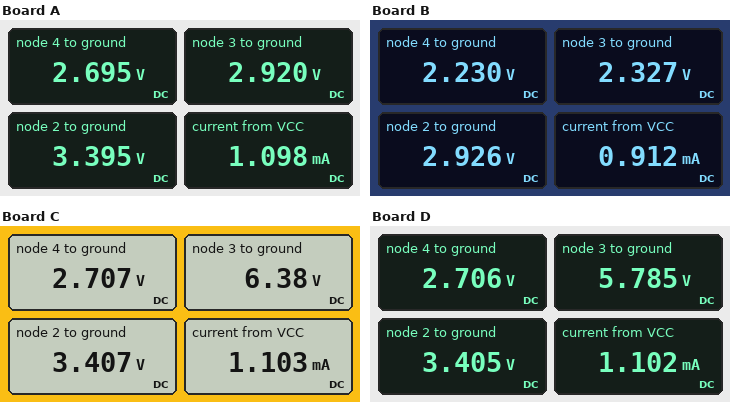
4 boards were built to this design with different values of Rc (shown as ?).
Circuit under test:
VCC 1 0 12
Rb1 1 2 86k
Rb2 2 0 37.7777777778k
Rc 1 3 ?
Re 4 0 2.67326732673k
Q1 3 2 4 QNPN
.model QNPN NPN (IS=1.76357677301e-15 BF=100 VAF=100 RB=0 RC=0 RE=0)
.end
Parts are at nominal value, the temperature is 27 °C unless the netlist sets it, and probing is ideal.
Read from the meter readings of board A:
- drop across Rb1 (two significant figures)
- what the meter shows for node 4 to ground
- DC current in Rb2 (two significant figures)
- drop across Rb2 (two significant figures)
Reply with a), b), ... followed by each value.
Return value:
a) 8.6 V
b) 2.695 V
c) 90 µA
d) 3.4 V
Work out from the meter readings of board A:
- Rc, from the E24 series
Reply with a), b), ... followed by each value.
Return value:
a) 9.1 kΩ
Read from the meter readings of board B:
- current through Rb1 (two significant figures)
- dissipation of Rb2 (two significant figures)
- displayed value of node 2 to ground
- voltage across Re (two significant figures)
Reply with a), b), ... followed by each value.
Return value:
a) 110 µA
b) 230 µW
c) 2.926 V
d) 2.2 V
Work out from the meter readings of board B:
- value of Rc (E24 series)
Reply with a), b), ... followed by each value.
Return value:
a) 12 kΩ
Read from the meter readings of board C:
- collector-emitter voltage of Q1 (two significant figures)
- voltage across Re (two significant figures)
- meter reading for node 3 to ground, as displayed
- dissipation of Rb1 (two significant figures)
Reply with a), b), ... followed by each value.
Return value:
a) 3.7 V
b) 2.7 V
c) 6.38 V
d) 860 µW
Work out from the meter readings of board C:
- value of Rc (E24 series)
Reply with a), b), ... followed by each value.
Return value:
a) 5.6 kΩ
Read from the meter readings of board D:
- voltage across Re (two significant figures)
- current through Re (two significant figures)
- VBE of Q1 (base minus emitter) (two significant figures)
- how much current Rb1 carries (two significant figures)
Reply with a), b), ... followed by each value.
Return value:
a) 2.7 V
b) 1.0 mA
c) 700 mV
d) 100 µA
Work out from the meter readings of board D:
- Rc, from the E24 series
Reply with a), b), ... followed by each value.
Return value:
a) 6.2 kΩ
